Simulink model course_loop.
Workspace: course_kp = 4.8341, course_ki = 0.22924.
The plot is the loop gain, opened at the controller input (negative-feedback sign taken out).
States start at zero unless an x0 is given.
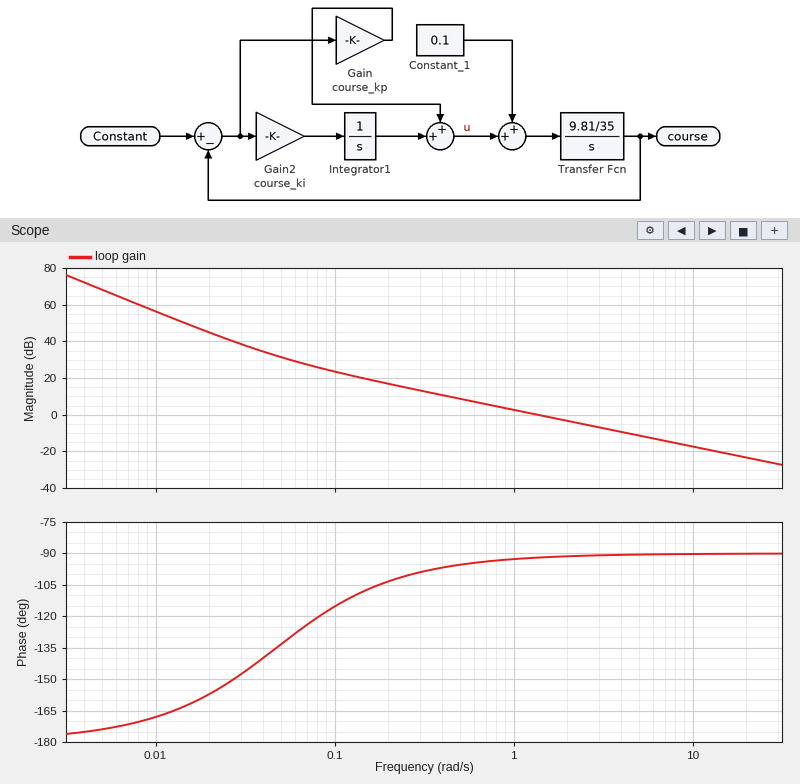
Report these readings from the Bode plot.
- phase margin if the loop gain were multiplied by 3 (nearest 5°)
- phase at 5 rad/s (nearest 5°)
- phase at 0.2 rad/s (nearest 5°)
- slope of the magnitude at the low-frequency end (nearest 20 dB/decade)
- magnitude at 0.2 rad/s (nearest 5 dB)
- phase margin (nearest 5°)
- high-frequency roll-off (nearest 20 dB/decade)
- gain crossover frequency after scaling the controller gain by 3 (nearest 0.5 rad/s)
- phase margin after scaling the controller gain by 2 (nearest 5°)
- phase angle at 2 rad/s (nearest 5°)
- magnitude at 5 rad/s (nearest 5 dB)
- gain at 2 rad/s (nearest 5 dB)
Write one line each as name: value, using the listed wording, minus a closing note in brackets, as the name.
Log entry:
phase margin if the loop gain were multiplied by 3: 90°
phase at 5 rad/s: -90°
phase at 0.2 rad/s: -105°
slope of the magnitude at the low-frequency end: -40 dB/decade
magnitude at 0.2 rad/s: 15 dB
phase margin: 90°
high-frequency roll-off: -20 dB/decade
gain crossover frequency after scaling the controller gain by 3: 4.0 rad/s
phase margin after scaling the controller gain by 2: 90°
phase angle at 2 rad/s: -90°
magnitude at 5 rad/s: -10 dB
gain at 2 rad/s: -5 dB
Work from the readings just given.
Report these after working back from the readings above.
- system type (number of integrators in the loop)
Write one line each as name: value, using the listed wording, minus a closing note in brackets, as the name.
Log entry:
system type: 2
